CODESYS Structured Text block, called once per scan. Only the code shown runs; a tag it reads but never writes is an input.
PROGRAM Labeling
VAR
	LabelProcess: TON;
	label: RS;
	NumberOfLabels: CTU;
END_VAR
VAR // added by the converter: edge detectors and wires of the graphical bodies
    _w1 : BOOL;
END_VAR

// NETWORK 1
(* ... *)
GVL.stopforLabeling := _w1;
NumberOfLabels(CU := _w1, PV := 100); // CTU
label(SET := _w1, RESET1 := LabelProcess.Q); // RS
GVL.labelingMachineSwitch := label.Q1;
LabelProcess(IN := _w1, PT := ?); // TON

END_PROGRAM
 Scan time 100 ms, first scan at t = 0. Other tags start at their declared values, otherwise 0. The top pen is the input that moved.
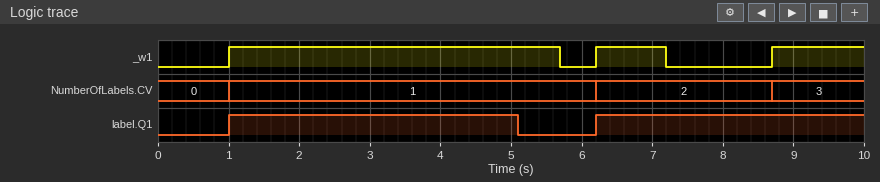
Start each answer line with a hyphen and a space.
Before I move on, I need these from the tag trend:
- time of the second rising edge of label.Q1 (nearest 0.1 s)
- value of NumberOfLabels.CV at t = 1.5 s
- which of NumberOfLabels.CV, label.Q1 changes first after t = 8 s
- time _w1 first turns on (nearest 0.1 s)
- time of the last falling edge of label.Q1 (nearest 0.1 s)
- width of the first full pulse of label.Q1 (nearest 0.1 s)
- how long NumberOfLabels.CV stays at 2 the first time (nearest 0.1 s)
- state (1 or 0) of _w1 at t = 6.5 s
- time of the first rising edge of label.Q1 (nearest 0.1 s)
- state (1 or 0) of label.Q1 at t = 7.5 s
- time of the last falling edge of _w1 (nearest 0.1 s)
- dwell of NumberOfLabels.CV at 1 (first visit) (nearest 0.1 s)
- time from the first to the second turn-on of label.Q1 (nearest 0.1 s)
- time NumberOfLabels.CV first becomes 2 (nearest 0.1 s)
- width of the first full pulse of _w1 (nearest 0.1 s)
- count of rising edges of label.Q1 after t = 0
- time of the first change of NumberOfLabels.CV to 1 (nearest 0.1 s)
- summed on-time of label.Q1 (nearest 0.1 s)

- 6.2 s
- 1
- NumberOfLabels.CV
- 1.0 s
- 5.1 s
- 4.1 s
- 2.5 s
- 1
- 1.0 s
- 1
- 7.2 s
- 5.2 s
- 5.2 s
- 6.2 s
- 4.7 s
- 2
- 1.0 s
- 7.9 s
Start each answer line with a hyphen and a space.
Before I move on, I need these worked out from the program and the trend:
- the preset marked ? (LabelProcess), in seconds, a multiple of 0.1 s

- 4.0 s
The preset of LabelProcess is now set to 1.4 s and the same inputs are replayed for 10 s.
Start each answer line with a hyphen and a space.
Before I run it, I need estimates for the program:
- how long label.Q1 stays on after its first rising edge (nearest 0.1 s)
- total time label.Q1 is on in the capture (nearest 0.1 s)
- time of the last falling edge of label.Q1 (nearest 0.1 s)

- 1.5 s
- 5.3 s
- 2.5 s
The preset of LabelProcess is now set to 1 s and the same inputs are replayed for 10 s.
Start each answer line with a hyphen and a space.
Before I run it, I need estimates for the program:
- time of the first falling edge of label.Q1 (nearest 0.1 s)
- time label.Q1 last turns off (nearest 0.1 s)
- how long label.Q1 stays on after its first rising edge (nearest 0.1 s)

- 2.1 s
- 9.8 s
- 1.1 s
